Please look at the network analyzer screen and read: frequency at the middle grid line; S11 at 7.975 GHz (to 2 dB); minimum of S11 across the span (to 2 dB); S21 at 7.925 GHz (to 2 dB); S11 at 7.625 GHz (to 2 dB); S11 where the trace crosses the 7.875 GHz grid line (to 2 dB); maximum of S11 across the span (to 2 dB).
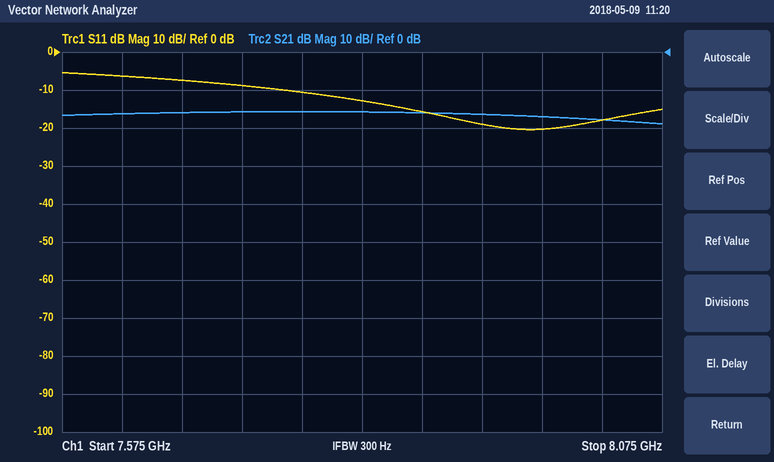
7.825 GHz
-20 dB
-20 dB
-16 dB
-6 dB
-16 dB
-6 dB
